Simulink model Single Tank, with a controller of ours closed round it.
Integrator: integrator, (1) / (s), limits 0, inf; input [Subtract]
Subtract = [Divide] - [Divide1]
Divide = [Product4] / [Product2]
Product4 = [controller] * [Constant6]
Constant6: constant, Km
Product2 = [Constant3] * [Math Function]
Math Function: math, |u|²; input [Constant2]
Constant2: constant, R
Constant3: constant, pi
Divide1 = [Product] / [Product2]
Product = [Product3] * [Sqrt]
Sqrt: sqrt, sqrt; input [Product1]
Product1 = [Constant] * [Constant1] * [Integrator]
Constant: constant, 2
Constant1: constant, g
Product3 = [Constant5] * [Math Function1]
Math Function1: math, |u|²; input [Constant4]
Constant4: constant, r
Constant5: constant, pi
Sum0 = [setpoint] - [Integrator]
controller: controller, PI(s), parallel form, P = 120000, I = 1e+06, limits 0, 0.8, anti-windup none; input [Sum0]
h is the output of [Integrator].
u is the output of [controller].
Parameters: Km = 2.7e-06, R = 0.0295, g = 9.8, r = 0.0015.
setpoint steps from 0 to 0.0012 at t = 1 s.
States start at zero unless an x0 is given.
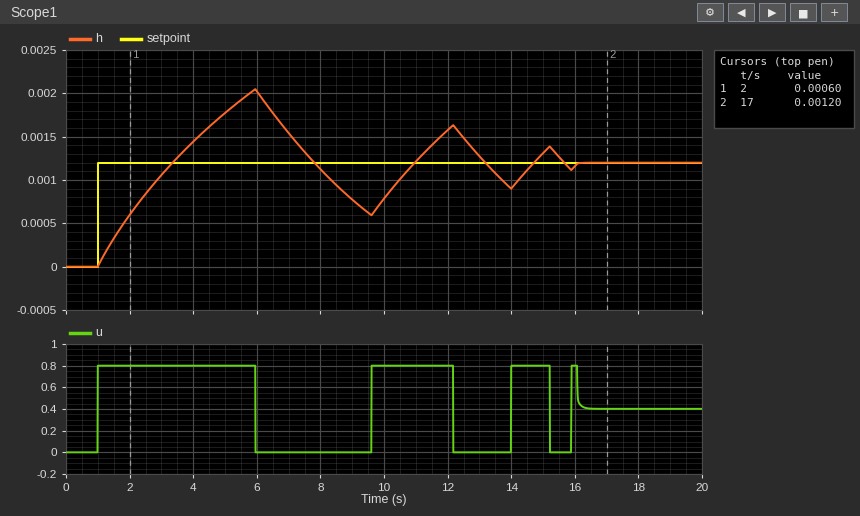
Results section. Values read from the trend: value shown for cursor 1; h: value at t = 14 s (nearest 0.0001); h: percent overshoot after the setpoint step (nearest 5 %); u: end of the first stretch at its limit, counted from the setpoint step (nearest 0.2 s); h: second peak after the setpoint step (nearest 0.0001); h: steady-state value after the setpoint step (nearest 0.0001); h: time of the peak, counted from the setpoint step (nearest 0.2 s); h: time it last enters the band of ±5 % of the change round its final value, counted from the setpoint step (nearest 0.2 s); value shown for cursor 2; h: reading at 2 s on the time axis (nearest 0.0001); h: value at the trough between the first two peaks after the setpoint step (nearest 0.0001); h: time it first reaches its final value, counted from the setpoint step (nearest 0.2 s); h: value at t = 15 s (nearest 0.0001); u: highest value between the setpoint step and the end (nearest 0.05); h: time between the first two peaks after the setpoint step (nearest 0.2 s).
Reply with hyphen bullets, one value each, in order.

- 0.00060
- 0.0009
- 70 %
- 5.0 s
- 0.0016
- 0.0012
- 5.0 s
- 15.0 s
- 0.00120
- 0.0006
- 0.0006
- 2.4 s
- 0.0013
- 0.80
- 6.2 s
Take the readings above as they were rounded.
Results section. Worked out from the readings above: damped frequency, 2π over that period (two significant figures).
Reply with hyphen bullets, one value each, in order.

- 1.0 rad/s
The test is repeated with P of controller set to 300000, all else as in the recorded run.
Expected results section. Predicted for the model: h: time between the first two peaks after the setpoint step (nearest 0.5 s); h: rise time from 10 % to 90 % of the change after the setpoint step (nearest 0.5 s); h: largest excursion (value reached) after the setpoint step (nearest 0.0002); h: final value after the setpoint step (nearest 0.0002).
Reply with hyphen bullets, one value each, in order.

- 4.5 s
- 2.0 s
- 0.0020
- 0.0012
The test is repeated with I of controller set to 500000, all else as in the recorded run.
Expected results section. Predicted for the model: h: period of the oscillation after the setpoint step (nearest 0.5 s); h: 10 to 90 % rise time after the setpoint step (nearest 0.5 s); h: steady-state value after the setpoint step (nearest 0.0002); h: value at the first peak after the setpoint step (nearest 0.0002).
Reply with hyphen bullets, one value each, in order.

- 5.0 s
- 2.0 s
- 0.0012
- 0.0020
